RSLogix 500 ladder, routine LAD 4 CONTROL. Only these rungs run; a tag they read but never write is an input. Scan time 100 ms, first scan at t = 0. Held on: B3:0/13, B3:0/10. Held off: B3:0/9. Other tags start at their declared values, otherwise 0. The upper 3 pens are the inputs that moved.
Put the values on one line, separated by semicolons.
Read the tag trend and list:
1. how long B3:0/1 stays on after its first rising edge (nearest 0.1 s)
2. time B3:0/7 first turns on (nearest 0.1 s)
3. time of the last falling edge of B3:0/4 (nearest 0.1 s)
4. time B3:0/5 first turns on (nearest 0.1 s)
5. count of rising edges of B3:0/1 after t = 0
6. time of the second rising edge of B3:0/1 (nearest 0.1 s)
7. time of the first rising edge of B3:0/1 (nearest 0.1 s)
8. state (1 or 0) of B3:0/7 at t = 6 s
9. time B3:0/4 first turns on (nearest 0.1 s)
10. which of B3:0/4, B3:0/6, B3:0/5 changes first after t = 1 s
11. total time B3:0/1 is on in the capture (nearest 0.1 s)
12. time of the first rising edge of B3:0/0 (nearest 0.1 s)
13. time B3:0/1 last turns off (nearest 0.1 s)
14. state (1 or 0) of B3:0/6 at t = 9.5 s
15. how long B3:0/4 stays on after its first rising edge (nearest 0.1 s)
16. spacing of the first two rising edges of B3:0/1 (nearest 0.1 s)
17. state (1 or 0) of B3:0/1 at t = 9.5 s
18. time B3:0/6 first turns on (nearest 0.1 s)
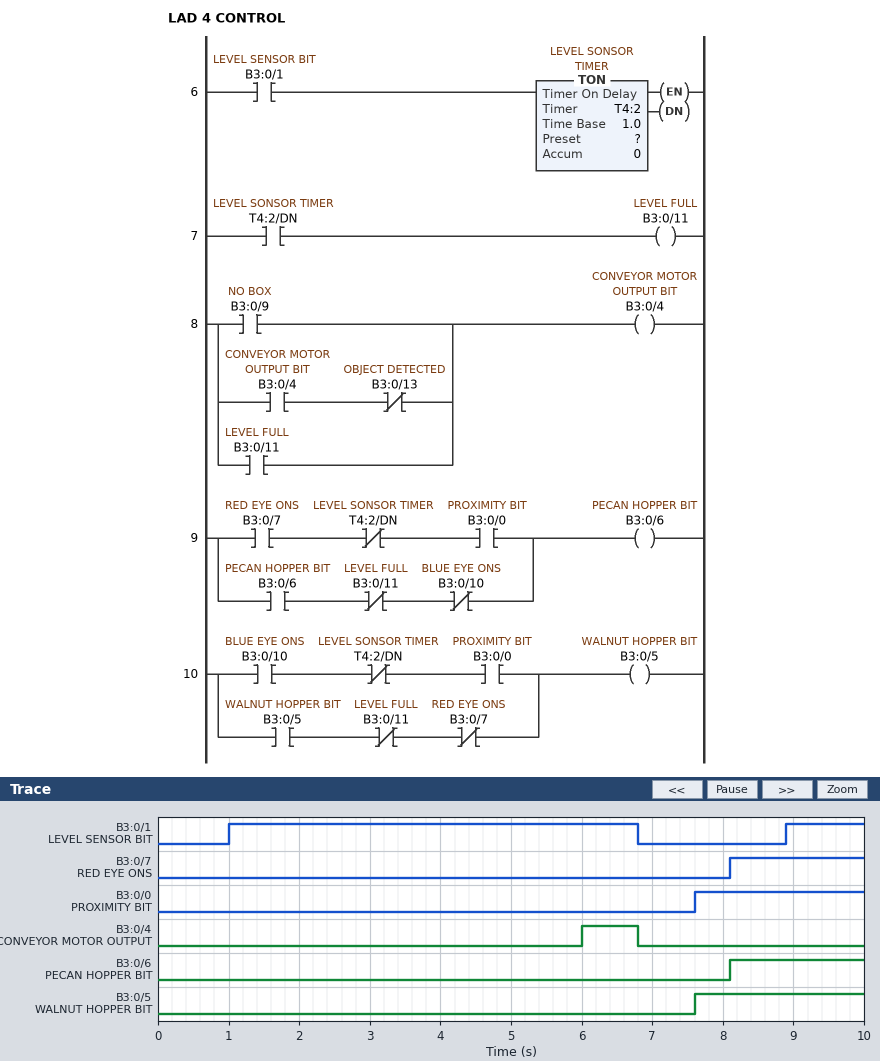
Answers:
5.8 s; 8.1 s; 6.8 s; 7.6 s; 2; 8.9 s; 1.0 s; 0; 6.0 s; B3:0/4; 6.9 s; 7.6 s; 6.8 s; 1; 0.8 s; 7.9 s; 1; 8.1 s
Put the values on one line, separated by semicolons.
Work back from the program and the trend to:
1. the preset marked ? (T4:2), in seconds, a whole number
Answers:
5 s
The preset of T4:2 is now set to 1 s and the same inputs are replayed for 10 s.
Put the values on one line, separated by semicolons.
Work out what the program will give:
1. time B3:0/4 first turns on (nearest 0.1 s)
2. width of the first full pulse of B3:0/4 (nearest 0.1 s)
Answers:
2.0 s; 4.8 s
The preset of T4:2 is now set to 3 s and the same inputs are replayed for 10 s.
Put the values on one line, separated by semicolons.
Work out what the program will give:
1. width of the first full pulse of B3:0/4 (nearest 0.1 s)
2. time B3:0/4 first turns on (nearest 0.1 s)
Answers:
2.8 s; 4.0 s
